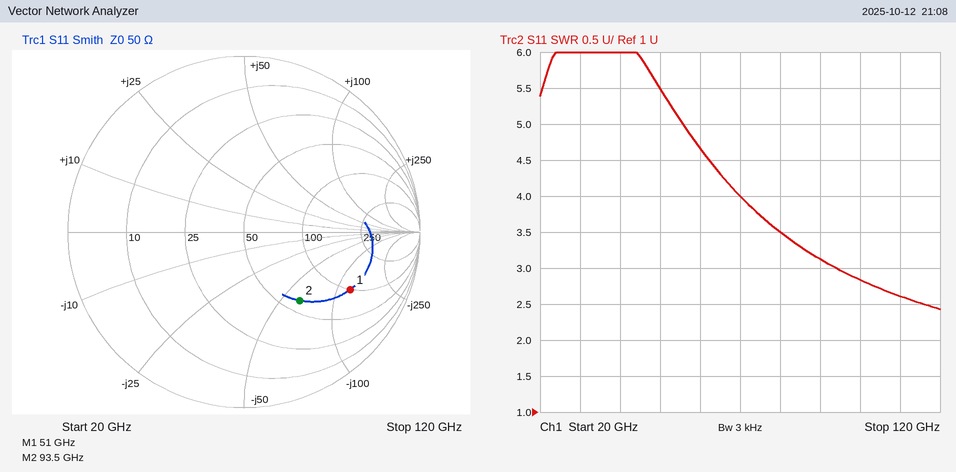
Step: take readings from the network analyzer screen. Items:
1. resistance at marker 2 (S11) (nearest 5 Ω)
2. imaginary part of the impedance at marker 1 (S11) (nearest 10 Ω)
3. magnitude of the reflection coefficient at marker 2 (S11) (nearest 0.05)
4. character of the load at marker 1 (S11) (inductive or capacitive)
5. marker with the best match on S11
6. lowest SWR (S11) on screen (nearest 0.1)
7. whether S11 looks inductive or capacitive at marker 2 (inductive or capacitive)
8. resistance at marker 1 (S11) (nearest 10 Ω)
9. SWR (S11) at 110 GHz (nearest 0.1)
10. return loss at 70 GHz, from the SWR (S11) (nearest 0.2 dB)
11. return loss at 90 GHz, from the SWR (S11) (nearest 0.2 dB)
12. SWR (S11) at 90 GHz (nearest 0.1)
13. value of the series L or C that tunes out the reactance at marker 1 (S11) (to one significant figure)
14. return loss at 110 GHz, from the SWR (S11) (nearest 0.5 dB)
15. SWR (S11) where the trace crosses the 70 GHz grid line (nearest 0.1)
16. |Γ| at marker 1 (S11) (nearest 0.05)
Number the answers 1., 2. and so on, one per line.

1. 60 Ω
2. -120 Ω
3. 0.50
4. capacitive
5. marker 2
6. 2.4
7. capacitive
8. 100 Ω
9. 2.6
10. 4.4 dB
11. 5.8 dB
12. 3.1
13. 400 pH
14. 7.0 dB
15. 4.0
16. 0.70
